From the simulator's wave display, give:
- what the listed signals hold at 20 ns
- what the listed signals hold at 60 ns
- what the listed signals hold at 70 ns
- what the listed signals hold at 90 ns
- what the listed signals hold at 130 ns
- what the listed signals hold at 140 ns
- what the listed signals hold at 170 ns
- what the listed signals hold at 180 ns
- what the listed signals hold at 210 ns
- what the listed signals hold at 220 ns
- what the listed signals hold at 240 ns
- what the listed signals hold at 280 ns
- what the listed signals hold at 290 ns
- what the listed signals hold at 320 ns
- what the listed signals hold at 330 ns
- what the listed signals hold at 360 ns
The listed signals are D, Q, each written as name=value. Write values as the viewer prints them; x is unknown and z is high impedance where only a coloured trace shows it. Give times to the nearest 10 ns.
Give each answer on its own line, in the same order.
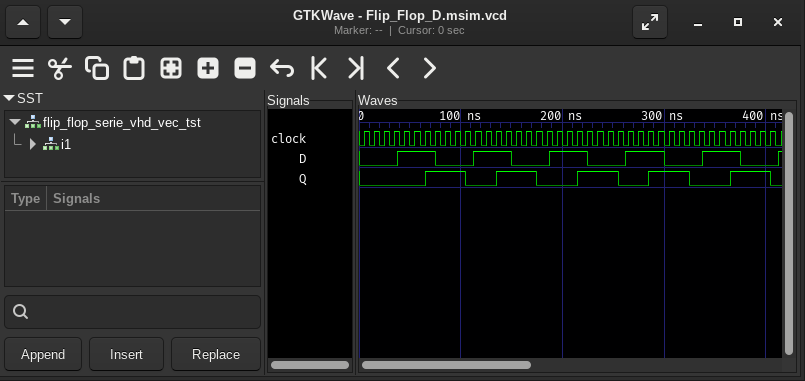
D=0, Q=0
D=1, Q=0
D=1, Q=1
D=0, Q=1
D=1, Q=0
D=1, Q=1
D=0, Q=1
D=0, Q=0
D=1, Q=0
D=1, Q=1
D=0, Q=1
D=1, Q=0
D=1, Q=1
D=0, Q=1
D=0, Q=0
D=1, Q=0
